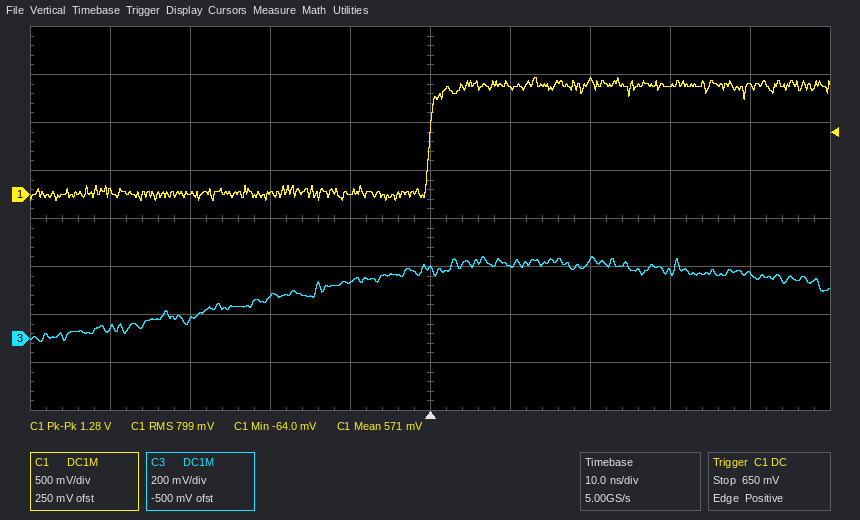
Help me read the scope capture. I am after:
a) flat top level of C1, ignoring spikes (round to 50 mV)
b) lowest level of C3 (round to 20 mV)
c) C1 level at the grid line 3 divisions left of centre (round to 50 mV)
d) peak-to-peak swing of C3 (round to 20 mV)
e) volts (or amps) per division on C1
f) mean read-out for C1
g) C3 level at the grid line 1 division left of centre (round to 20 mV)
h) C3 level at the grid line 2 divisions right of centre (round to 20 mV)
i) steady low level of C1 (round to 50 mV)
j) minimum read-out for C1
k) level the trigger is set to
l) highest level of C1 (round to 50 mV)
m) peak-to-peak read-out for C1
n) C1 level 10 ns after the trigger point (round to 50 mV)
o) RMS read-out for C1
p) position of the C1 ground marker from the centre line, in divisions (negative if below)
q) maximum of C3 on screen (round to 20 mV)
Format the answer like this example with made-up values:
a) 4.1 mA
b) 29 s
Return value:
a) 1.15 V
b) -20 mV
c) 0 mV
d) 360 mV
e) 500 mV
f) 571 mV
g) 240 mV
h) 320 mV
i) 0 mV
j) -64.0 mV
k) 650 mV
l) 1.20 V
m) 1.28 V
n) 1.15 V
o) 799 mV
p) +0.5 div
q) 340 mV
